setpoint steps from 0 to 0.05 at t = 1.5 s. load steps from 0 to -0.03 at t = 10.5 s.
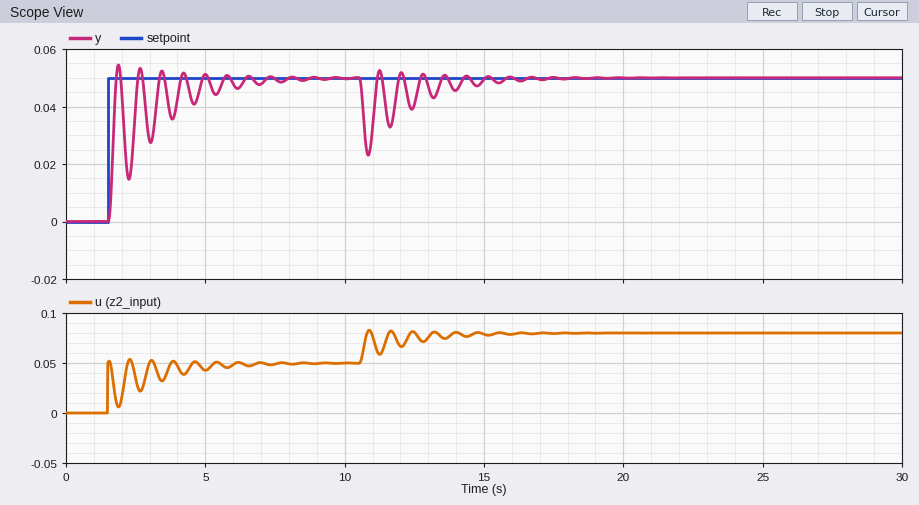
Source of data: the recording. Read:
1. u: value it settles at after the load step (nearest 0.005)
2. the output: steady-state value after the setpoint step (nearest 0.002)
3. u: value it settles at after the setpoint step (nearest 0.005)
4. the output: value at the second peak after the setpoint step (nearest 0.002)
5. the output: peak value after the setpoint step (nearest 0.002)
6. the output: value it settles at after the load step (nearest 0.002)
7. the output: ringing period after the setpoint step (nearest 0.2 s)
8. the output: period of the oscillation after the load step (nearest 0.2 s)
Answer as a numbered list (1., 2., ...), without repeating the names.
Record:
1. 0.080
2. 0.050
3. 0.050
4. 0.054
5. 0.054
6. 0.050
7. 0.8 s
8. 0.8 s
